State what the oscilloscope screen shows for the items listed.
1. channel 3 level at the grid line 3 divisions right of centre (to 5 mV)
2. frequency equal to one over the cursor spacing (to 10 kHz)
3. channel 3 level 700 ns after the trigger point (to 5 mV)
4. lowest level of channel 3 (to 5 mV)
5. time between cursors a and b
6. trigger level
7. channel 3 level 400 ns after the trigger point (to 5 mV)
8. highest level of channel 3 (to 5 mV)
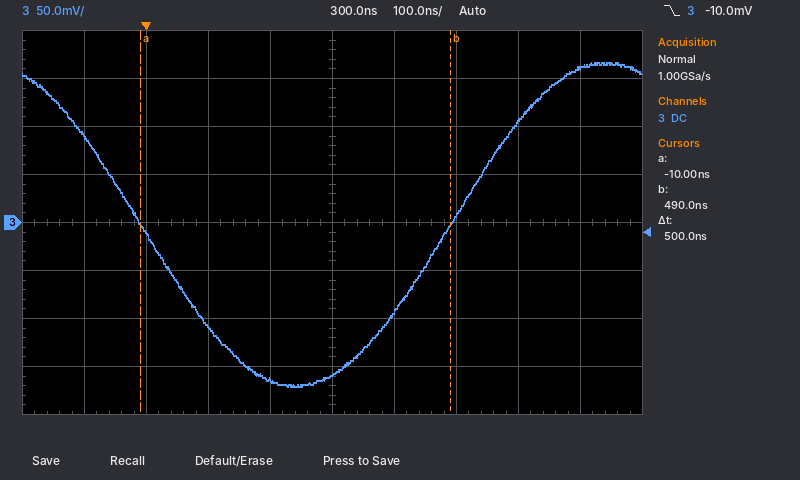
105 mV
2.00 MHz
160 mV
-170 mV
500 ns
-10.0 mV
-95 mV
165 mV
